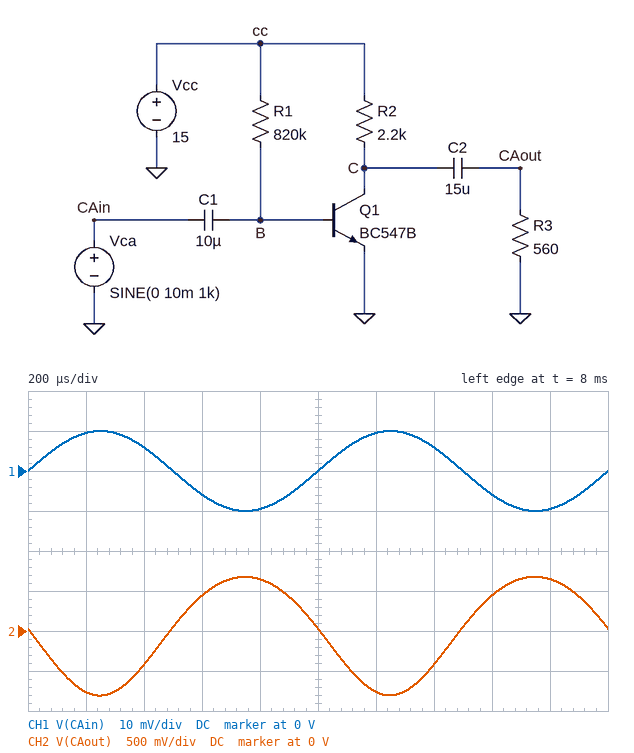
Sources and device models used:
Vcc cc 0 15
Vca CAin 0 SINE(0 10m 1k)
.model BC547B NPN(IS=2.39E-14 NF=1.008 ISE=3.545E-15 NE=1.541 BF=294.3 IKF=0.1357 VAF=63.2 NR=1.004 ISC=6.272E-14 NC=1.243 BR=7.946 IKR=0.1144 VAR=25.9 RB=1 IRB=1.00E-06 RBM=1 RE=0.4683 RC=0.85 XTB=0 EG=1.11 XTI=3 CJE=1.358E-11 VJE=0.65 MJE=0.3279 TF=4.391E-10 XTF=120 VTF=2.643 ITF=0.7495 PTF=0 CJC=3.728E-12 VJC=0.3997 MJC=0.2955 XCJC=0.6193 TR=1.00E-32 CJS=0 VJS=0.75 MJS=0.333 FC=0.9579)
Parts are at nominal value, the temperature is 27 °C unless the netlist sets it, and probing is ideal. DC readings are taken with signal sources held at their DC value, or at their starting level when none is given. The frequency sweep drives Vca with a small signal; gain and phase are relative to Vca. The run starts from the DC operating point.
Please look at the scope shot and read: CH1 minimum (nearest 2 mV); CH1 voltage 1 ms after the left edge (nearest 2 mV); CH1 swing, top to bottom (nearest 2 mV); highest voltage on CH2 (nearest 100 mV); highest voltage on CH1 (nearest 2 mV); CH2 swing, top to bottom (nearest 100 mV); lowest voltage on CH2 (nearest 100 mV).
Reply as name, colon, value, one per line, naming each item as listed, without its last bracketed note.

CH1 minimum: -10 mV
CH1 voltage 1 ms after the left edge: 0 V
CH1 swing, top to bottom: 20 mV
highest voltage on CH2: 700 mV
highest voltage on CH1: 10 mV
CH2 swing, top to bottom: 1.5 V
lowest voltage on CH2: -800 mV
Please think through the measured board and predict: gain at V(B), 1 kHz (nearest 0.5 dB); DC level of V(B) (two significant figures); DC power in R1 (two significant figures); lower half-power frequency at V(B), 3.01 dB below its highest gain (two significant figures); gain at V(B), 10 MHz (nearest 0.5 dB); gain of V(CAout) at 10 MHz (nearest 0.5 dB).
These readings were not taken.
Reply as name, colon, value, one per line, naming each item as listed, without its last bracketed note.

gain at V(B), 1 kHz: 0 dB
DC level of V(B): 680 mV
DC power in R1: 250 µW
lower half-power frequency at V(B), 3.01 dB below its highest gain: 9.8 Hz
gain at V(B), 10 MHz: 0 dB
gain of V(CAout) at 10 MHz: 37.5 dB
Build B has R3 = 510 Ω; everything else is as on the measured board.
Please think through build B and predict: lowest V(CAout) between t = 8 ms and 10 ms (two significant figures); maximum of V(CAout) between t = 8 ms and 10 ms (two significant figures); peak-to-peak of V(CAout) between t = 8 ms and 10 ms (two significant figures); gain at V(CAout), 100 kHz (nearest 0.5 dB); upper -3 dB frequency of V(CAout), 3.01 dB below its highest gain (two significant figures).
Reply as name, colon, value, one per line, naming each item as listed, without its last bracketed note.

lowest V(CAout) between t = 8 ms and 10 ms: -750 mV
maximum of V(CAout) between t = 8 ms and 10 ms: 630 mV
peak-to-peak of V(CAout) between t = 8 ms and 10 ms: 1.4 V
gain at V(CAout), 100 kHz: 37.0 dB
upper -3 dB frequency of V(CAout), 3.01 dB below its highest gain: 170 MHz
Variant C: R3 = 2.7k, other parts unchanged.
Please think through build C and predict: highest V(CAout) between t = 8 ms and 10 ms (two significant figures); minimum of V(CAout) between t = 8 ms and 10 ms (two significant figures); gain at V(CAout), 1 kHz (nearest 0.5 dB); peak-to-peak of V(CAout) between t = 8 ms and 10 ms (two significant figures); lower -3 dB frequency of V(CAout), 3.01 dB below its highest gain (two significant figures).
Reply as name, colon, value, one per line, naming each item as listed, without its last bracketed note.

highest V(CAout) between t = 8 ms and 10 ms: 1.8 V
minimum of V(CAout) between t = 8 ms and 10 ms: -2.1 V
gain at V(CAout), 1 kHz: 45.5 dB
peak-to-peak of V(CAout) between t = 8 ms and 10 ms: 3.8 V
lower -3 dB frequency of V(CAout), 3.01 dB below its highest gain: 10 Hz
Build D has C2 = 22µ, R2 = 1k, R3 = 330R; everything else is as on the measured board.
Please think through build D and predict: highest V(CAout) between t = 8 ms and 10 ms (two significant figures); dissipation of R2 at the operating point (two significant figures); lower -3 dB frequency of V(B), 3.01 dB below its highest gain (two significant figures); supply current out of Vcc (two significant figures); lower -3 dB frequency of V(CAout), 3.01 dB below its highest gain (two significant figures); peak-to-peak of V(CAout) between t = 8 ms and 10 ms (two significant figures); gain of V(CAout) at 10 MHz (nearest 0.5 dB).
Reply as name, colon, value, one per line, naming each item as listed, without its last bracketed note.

highest V(CAout) between t = 8 ms and 10 ms: 410 mV
dissipation of R2 at the operating point: 30 mW
lower -3 dB frequency of V(B), 3.01 dB below its highest gain: 9.7 Hz
supply current out of Vcc: 5.5 mA
lower -3 dB frequency of V(CAout), 3.01 dB below its highest gain: 12 Hz
peak-to-peak of V(CAout) between t = 8 ms and 10 ms: 900 mV
gain of V(CAout) at 10 MHz: 33.0 dB
